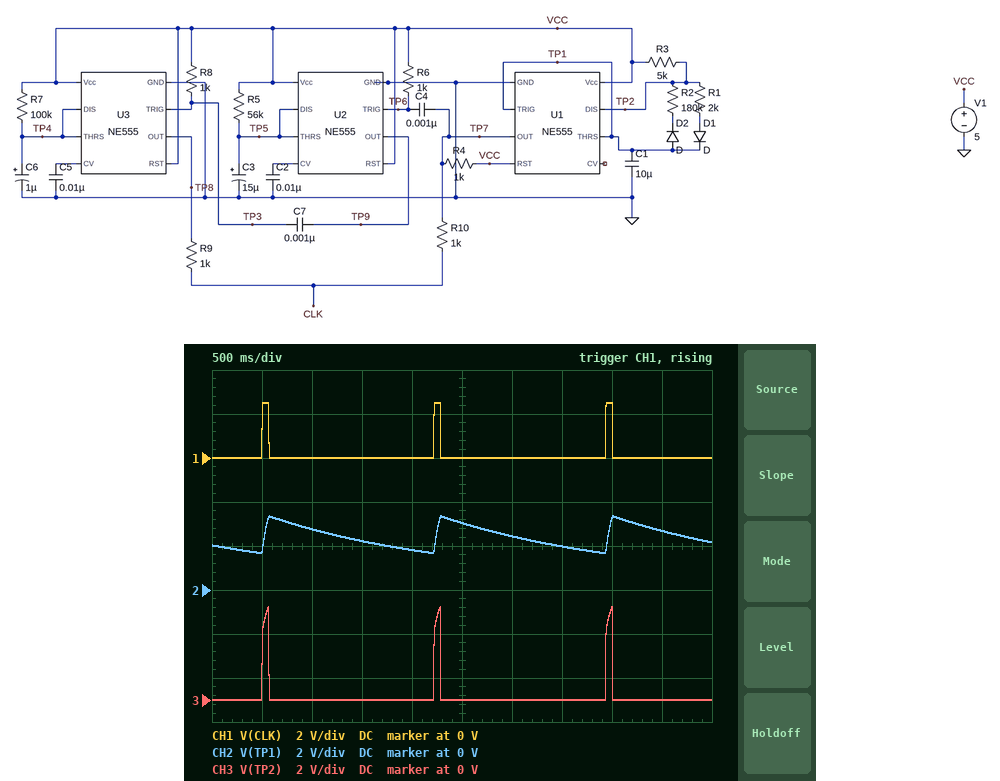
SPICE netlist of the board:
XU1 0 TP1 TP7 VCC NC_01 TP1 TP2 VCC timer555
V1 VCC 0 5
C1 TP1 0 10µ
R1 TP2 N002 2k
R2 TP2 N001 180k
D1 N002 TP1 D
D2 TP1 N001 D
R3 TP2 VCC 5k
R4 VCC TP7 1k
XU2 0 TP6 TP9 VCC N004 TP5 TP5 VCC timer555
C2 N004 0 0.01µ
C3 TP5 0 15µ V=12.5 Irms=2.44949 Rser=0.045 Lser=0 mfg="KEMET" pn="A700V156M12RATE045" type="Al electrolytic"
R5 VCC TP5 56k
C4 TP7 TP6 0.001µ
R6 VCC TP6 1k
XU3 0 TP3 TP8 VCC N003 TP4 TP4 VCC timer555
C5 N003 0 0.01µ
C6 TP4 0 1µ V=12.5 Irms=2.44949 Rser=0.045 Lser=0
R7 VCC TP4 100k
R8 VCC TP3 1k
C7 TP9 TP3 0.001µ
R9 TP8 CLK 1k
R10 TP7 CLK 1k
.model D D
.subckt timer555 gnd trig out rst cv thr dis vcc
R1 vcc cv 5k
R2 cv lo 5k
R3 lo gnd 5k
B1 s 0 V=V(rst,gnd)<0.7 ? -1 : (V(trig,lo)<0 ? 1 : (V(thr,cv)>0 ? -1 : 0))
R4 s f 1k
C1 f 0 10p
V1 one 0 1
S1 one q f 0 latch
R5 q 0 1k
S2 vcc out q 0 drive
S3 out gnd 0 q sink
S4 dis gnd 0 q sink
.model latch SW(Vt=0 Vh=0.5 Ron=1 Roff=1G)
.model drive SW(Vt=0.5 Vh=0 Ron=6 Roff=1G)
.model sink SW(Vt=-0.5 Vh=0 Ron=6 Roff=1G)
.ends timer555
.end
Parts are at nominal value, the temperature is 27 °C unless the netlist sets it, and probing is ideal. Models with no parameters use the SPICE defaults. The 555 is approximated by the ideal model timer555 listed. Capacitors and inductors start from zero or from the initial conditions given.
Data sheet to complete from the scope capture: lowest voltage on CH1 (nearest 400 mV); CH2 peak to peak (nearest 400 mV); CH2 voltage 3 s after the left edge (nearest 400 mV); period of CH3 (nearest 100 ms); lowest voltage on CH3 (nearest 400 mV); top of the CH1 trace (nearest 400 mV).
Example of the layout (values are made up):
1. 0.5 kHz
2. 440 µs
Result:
1. 0 V
2. 1.6 V
3. 2.4 V
4. 1.7 s
5. 0 V
6. 2.4 V
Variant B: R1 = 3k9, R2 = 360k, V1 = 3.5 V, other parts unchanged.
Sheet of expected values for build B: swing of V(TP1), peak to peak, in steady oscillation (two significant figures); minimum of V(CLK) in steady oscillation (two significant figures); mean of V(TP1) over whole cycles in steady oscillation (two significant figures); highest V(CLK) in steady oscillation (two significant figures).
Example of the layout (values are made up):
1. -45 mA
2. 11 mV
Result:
1. 1.2 V
2. 10 mV
3. 1.7 V
4. 1.8 V
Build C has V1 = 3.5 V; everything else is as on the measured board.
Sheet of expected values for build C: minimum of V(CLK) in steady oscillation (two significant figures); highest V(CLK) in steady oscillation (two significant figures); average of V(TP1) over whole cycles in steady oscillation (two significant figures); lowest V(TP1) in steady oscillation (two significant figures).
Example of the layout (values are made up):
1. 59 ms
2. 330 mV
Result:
1. 10 mV
2. 1.8 V
3. 1.7 V
4. 1.2 V
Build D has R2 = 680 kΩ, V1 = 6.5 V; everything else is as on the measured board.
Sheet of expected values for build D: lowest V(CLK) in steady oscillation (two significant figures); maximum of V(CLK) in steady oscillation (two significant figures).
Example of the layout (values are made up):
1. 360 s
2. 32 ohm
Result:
1. 19 mV
2. 3.3 V
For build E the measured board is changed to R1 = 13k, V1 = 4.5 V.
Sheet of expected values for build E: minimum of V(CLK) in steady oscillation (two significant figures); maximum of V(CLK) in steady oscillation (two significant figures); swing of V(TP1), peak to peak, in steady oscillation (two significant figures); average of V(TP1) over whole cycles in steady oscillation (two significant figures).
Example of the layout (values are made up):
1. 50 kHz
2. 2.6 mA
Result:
1. 13 mV
2. 2.3 V
3. 1.5 V
4. 2.2 V
